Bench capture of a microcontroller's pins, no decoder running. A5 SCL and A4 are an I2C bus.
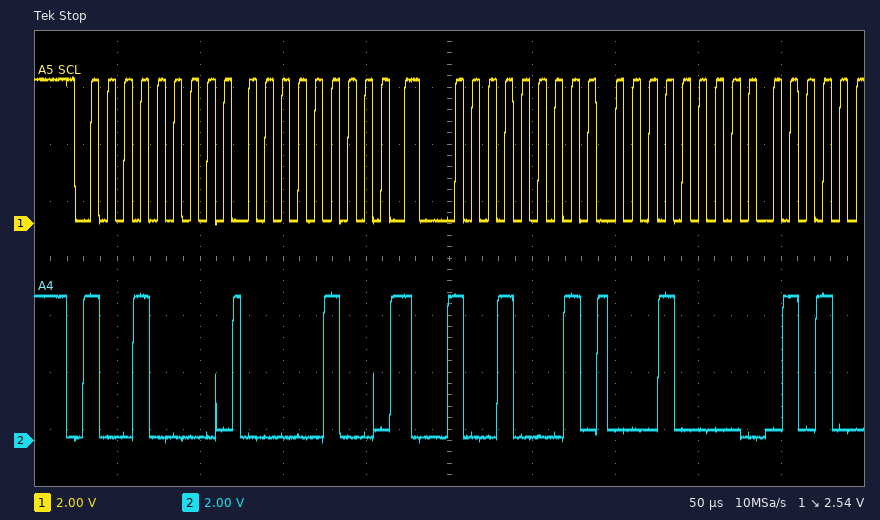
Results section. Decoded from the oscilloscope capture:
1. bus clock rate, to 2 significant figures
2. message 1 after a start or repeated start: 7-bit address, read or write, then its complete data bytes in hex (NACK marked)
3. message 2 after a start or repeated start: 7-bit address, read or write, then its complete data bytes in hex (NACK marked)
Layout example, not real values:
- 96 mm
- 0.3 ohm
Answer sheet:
- 100 kHz
- 0x48 write: 04
- 0x48 read: 10
